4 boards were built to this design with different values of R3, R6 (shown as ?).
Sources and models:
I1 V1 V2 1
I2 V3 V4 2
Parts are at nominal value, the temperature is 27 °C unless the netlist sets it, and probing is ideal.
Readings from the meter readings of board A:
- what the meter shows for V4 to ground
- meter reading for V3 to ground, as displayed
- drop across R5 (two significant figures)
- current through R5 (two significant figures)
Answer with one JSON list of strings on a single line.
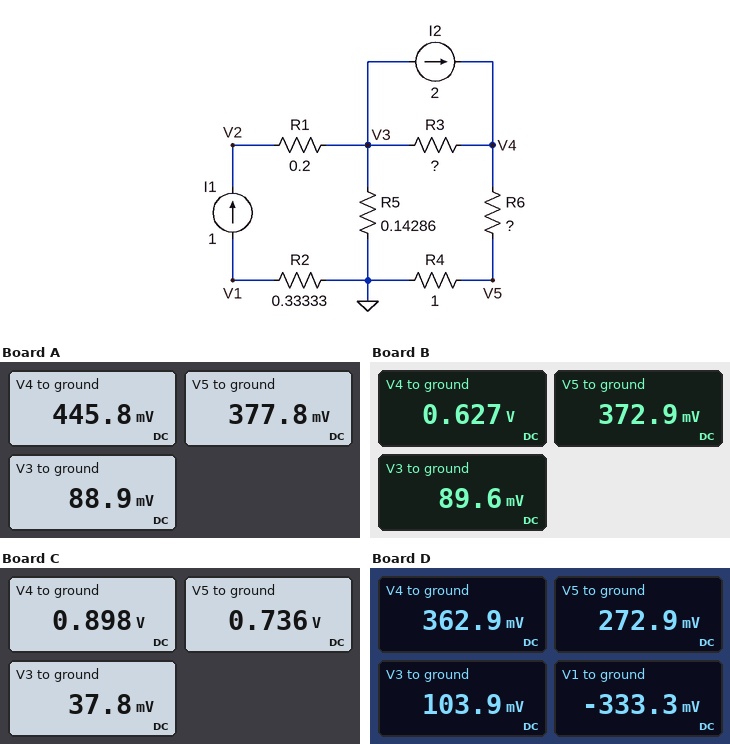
["445.8 mV", "88.9 mV", "89 mV", "620 mA"]
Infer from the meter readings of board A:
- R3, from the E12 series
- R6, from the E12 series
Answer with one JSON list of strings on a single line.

["0.22 Ω", "0.18 Ω"]
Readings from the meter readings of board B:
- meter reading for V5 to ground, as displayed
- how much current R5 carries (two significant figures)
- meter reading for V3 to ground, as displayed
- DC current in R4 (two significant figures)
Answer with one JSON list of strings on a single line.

["372.9 mV", "630 mA", "89.6 mV", "370 mA"]
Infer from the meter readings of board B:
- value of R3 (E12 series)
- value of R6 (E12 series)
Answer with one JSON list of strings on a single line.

["0.33 Ω", "0.68 Ω"]
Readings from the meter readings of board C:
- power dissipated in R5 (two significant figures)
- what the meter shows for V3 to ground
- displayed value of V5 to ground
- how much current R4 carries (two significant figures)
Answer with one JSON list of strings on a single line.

["10 mW", "37.8 mV", "0.736 V", "740 mA"]
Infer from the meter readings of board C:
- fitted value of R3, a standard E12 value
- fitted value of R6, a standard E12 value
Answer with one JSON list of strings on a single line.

["0.68 Ω", "0.22 Ω"]
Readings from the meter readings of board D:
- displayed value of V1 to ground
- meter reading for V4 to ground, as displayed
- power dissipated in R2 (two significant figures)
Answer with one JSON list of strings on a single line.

["-333.3 mV", "362.9 mV", "330 mW"]
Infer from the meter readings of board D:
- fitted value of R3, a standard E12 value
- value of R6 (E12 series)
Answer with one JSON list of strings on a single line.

["0.15 Ω", "0.33 Ω"]
